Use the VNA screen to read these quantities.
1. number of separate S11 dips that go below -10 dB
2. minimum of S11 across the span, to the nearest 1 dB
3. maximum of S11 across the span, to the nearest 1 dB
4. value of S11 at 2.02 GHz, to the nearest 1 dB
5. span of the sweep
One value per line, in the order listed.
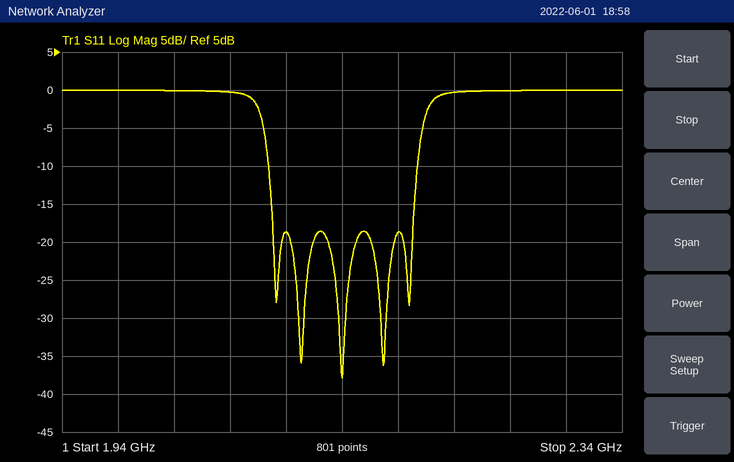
5
-38 dB
0 dB
0 dB
400 MHz
